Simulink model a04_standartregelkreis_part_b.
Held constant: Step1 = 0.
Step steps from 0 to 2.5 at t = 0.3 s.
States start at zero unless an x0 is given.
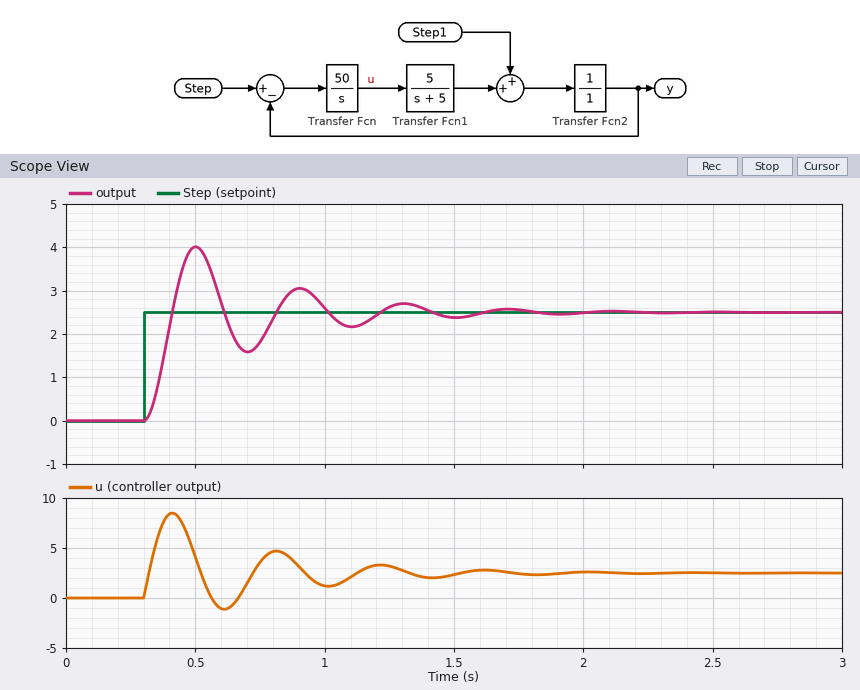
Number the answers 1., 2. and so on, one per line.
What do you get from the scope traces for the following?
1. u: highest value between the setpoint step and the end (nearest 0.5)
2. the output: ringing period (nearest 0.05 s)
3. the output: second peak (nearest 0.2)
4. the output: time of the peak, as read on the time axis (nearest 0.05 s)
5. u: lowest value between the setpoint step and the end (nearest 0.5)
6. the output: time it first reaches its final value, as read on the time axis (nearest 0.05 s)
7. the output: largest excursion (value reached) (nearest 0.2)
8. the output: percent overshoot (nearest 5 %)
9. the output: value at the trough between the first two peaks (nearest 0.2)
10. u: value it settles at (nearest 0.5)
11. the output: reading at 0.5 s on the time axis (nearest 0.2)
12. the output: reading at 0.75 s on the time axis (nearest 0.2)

1. 8.5
2. 0.40 s
3. 3.0
4. 0.50 s
5. -1.0
6. 0.40 s
7. 4.0
8. 60 %
9. 1.6
10. 2.5
11. 4.0
12. 1.8
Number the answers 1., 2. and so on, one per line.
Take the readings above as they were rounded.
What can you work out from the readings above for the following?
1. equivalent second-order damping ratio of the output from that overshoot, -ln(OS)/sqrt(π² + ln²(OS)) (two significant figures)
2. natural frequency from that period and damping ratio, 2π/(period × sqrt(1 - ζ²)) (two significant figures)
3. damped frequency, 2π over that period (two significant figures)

1. 0.16
2. 16 rad/s
3. 16 rad/s
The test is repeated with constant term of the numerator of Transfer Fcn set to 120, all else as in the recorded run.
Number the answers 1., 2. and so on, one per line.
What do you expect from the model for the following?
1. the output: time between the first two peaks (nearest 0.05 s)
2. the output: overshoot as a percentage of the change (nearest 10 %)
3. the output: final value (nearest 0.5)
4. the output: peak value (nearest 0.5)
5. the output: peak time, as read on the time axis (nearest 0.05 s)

1. 0.25 s
2. 70 %
3. 2.5
4. 4.5
5. 0.45 s
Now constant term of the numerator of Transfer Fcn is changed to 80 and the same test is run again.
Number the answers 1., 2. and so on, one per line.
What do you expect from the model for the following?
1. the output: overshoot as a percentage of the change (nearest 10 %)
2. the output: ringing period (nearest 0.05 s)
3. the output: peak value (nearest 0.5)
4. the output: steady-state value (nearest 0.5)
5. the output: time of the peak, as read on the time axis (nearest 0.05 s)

1. 70 %
2. 0.30 s
3. 4.0
4. 2.5
5. 0.45 s
